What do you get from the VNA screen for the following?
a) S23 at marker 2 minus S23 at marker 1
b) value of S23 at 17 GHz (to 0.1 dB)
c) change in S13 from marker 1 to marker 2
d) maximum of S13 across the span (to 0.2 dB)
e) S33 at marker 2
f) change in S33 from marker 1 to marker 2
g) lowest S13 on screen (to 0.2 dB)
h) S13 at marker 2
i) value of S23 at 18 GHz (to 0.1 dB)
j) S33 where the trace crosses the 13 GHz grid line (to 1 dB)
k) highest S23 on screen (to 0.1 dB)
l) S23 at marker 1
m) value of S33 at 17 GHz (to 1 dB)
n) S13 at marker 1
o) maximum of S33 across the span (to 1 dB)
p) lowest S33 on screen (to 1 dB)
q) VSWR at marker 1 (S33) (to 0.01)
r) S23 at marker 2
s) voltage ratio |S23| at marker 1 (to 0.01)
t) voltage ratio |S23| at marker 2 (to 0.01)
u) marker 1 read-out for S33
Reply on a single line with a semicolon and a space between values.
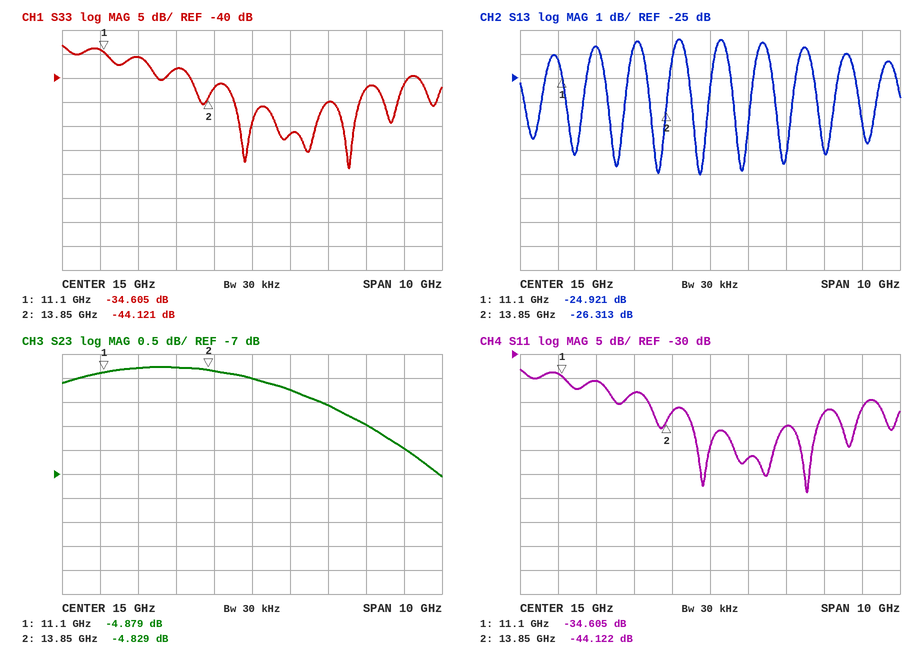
0.050 dB; -5.6 dB; -1.392 dB; -23.4 dB; -44.121 dB; -9.516 dB; -29.0 dB; -26.313 dB; -6.0 dB; -38 dB; -4.8 dB; -4.879 dB; -45 dB; -24.921 dB; -33 dB; -59 dB; 1.04; -4.829 dB; 0.57; 0.57; -34.605 dB
